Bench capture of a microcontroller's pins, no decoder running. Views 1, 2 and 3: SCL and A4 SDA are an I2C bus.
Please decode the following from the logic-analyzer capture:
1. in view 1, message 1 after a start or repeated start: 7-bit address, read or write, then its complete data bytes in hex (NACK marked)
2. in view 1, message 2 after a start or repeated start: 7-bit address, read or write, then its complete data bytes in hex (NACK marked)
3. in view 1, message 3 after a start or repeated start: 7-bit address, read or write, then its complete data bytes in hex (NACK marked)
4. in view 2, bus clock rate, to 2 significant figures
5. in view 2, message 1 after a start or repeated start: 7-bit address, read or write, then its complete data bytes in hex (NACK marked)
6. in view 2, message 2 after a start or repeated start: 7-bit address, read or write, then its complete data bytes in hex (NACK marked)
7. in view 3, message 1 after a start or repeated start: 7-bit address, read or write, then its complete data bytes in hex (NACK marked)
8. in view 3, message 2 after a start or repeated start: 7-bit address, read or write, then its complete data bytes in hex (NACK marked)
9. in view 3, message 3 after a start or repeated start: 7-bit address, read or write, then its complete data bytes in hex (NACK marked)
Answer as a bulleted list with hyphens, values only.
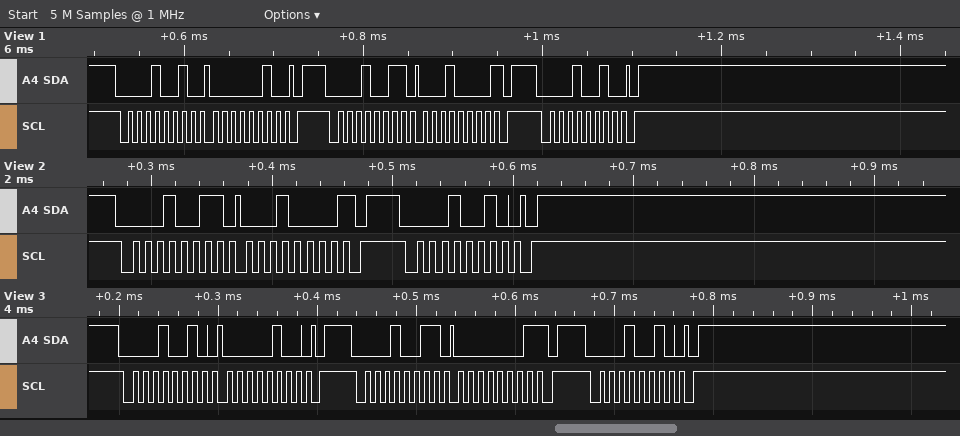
- 0x09 write: 02
- 0x09 read: 10 NACK
- 0x09 write
- 100 kHz
- 0x09 read: 10 NACK
- 0x09 write
- 0x09 write: 04
- 0x09 read: 01 NACK
- 0x09 write
